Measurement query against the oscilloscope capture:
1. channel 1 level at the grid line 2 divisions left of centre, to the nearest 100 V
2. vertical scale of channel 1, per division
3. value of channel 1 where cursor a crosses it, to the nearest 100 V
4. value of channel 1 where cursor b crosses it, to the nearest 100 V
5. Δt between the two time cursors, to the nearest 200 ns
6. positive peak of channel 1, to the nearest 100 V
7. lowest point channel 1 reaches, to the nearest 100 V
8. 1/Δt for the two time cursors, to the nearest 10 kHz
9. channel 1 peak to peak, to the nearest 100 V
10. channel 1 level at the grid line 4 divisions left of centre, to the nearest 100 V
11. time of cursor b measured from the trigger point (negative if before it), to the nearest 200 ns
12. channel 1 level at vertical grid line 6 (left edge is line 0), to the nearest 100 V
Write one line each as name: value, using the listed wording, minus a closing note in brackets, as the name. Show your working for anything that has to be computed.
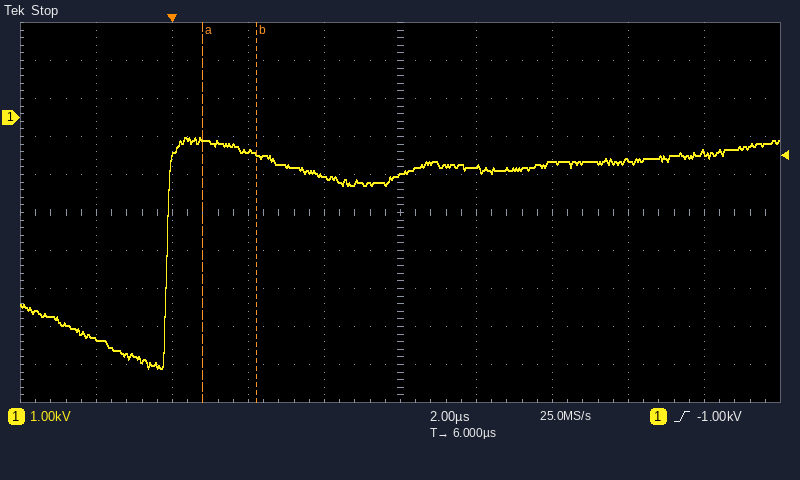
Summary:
channel 1 level at the grid line 2 divisions left of centre, to the nearest 100 V: -900 V
vertical scale of channel 1, per division: 1 kV
value of channel 1 where cursor a crosses it, to the nearest 100 V: -600 V
value of channel 1 where cursor b crosses it, to the nearest 100 V: -1.0 kV
Δt between the two time cursors, to the nearest 200 ns: 1.4 µs
positive peak of channel 1, to the nearest 100 V: -500 V
lowest point channel 1 reaches, to the nearest 100 V: -6.6 kV
1/Δt for the two time cursors, to the nearest 10 kHz: 1 / 1.4 µs ≈ 710 kHz
channel 1 peak to peak, to the nearest 100 V: -500 V − (-6.6 kV) = 6.1 kV
channel 1 level at the grid line 4 divisions left of centre, to the nearest 100 V: -5.8 kV
time of cursor b measured from the trigger point (negative if before it), to the nearest 200 ns: +2.2 µs
channel 1 level at vertical grid line 6 (left edge is line 0), to the nearest 100 V: -1.3 kV
